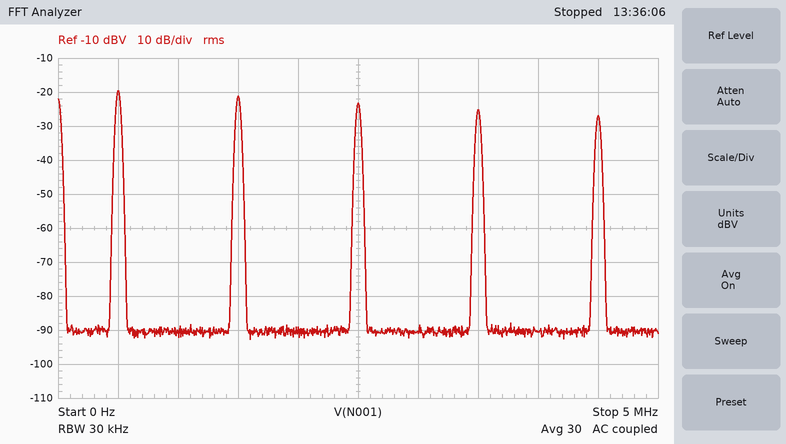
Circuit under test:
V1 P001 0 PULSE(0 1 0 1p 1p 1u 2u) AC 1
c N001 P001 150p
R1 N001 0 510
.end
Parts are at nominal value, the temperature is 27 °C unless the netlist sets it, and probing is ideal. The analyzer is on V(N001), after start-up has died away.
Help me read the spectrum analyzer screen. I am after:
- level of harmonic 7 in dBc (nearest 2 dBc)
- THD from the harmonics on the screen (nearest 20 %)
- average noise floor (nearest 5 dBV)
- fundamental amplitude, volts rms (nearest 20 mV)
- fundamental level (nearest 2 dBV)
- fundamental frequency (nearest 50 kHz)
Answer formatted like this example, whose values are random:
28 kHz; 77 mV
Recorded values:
-6 dBc; 120 %; -90 dBV; 100 mV; -20 dBV; 500 kHz
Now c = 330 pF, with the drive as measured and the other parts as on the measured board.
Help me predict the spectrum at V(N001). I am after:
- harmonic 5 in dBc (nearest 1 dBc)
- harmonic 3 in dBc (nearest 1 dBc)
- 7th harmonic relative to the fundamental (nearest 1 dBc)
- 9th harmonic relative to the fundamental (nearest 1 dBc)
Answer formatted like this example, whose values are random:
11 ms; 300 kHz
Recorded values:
-8 dBc; -4 dBc; -11 dBc; -13 dBc
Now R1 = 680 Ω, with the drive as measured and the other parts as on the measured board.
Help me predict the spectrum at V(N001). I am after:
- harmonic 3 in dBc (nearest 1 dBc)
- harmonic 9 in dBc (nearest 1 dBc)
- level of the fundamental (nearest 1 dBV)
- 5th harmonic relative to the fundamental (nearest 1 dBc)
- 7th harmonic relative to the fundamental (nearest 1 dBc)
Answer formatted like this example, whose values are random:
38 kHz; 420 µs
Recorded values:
-2 dBc; -9 dBc; -17 dBV; -5 dBc; -7 dBc
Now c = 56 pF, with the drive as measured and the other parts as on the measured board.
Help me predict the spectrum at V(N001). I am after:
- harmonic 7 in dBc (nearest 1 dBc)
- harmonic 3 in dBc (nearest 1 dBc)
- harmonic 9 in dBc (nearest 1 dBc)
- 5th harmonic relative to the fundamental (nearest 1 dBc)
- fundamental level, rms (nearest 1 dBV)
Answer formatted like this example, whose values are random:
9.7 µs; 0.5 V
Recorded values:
-1 dBc; 0 dBc; -2 dBc; -1 dBc; -28 dBV
